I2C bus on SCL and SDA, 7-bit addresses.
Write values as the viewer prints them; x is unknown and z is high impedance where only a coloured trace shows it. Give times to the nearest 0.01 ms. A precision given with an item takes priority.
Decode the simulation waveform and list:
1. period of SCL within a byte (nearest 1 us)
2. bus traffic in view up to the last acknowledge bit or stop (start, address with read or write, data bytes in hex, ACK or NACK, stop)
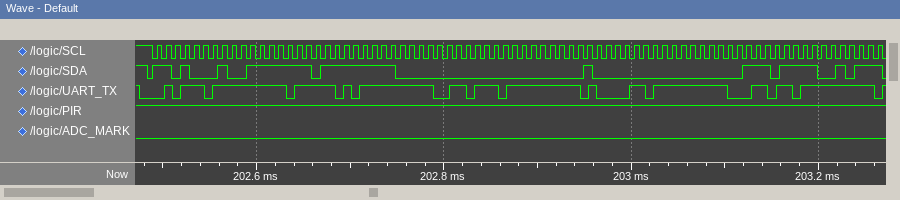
10 us
start, address 68 read ACK, 7F ACK, FF ACK, 00 ACK, 00 ACK, 40 ACK, 00 ACK, EF ACK
